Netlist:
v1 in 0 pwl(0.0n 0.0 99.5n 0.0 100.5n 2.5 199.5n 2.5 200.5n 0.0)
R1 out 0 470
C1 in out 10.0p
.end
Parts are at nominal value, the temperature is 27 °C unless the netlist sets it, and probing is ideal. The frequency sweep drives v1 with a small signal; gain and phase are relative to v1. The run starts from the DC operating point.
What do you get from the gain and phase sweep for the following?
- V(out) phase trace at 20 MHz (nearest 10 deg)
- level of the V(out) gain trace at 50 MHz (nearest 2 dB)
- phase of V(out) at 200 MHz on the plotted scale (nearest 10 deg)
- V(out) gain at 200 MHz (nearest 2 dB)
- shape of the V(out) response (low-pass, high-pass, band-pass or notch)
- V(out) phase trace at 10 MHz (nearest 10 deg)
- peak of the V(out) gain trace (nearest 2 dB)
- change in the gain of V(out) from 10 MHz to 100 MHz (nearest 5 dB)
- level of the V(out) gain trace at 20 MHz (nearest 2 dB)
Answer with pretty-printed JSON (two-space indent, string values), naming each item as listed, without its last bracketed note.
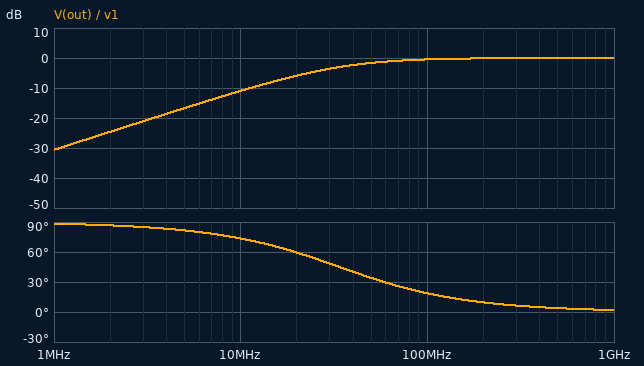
{
  "V(out) phase trace at 20 MHz": "60 deg",
  "level of the V(out) gain trace at 50 MHz": "-2 dB",
  "phase of V(out) at 200 MHz on the plotted scale": "10 deg",
  "V(out) gain at 200 MHz": "0 dB",
  "shape of the V(out) response": "high-pass",
  "V(out) phase trace at 10 MHz": "70 deg",
  "peak of the V(out) gain trace": "0 dB",
  "change in the gain of V(out) from 10 MHz to 100 MHz": "10 dB",
  "level of the V(out) gain trace at 20 MHz": "-6 dB"
}
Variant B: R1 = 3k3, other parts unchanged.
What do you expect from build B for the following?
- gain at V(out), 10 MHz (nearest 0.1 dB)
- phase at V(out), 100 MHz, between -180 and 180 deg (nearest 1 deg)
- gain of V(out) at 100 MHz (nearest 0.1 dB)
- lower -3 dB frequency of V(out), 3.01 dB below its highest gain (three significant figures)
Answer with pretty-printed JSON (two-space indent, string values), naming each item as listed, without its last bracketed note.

{
  "gain at V(out), 10 MHz": "-0.9 dB",
  "phase at V(out), 100 MHz, between -180 and 180 deg": "3 deg",
  "gain of V(out) at 100 MHz": "0 dB",
  "lower -3 dB frequency of V(out), 3.01 dB below its highest gain": "4.82 MHz"
}
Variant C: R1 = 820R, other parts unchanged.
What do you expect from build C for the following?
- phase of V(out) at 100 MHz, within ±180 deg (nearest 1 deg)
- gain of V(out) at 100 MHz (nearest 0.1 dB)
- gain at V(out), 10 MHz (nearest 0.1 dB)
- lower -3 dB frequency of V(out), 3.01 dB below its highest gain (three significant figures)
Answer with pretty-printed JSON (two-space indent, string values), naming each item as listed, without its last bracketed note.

{
  "phase of V(out) at 100 MHz, within ±180 deg": "11 deg",
  "gain of V(out) at 100 MHz": "-0.2 dB",
  "gain at V(out), 10 MHz": "-6.8 dB",
  "lower -3 dB frequency of V(out), 3.01 dB below its highest gain": "19.4 MHz"
}
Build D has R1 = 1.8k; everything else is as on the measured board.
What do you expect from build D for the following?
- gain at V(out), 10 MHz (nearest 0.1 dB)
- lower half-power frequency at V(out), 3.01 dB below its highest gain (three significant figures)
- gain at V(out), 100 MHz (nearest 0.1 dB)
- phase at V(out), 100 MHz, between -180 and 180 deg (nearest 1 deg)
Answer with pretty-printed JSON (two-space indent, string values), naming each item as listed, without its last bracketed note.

{
  "gain at V(out), 10 MHz": "-2.5 dB",
  "lower half-power frequency at V(out), 3.01 dB below its highest gain": "8.84 MHz",
  "gain at V(out), 100 MHz": "0 dB",
  "phase at V(out), 100 MHz, between -180 and 180 deg": "5 deg"
}
